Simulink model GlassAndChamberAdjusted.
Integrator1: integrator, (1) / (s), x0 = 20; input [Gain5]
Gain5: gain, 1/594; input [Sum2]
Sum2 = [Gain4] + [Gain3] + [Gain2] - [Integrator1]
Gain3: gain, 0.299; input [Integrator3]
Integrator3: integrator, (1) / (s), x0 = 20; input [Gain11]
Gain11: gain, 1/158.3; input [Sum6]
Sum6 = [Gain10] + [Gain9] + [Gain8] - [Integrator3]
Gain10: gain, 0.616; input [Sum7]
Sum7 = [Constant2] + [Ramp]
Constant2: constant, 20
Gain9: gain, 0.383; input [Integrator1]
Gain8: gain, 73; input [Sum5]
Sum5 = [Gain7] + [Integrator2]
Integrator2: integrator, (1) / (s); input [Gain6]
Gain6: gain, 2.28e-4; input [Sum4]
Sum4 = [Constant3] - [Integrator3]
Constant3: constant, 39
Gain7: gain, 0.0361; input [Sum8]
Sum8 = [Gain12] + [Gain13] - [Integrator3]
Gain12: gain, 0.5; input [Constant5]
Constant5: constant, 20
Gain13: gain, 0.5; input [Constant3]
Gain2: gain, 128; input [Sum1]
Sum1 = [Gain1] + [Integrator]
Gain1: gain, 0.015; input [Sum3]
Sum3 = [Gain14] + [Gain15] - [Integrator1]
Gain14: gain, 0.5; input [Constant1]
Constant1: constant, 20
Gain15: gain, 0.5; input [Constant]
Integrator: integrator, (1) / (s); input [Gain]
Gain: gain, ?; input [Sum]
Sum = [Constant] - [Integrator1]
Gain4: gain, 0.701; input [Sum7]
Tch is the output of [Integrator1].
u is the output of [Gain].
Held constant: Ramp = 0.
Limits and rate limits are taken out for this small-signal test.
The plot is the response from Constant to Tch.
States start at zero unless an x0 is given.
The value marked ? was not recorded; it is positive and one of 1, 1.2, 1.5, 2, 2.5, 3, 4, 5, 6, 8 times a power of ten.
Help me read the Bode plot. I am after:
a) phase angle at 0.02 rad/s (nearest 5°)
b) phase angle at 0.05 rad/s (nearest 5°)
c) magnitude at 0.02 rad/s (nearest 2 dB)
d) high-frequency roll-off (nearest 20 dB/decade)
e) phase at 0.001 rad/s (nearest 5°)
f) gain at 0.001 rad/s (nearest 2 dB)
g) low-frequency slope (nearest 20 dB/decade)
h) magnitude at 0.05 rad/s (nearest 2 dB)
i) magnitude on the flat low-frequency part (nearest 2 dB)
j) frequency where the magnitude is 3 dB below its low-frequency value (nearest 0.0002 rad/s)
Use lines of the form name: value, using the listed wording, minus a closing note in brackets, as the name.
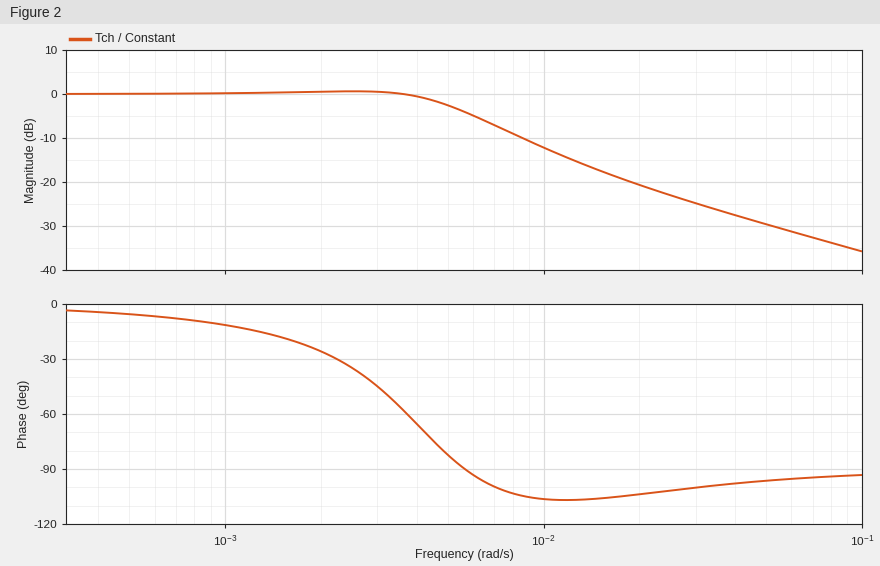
phase angle at 0.02 rad/s: -105°
phase angle at 0.05 rad/s: -95°
magnitude at 0.02 rad/s: -20 dB
high-frequency roll-off: -20 dB/decade
phase at 0.001 rad/s: -10°
gain at 0.001 rad/s: 0 dB
low-frequency slope: 0 dB/decade
magnitude at 0.05 rad/s: -30 dB
magnitude on the flat low-frequency part: 0 dB
frequency where the magnitude is 3 dB below its low-frequency value: 0.0052 rad/s
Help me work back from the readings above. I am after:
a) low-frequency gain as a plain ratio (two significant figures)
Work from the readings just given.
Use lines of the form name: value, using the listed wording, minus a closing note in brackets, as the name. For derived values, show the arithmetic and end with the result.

low-frequency gain as a plain ratio: 10^(0 / 20) = 1.0
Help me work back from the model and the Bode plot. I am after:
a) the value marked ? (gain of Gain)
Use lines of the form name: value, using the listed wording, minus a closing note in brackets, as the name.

the value marked ?: 8e-05
